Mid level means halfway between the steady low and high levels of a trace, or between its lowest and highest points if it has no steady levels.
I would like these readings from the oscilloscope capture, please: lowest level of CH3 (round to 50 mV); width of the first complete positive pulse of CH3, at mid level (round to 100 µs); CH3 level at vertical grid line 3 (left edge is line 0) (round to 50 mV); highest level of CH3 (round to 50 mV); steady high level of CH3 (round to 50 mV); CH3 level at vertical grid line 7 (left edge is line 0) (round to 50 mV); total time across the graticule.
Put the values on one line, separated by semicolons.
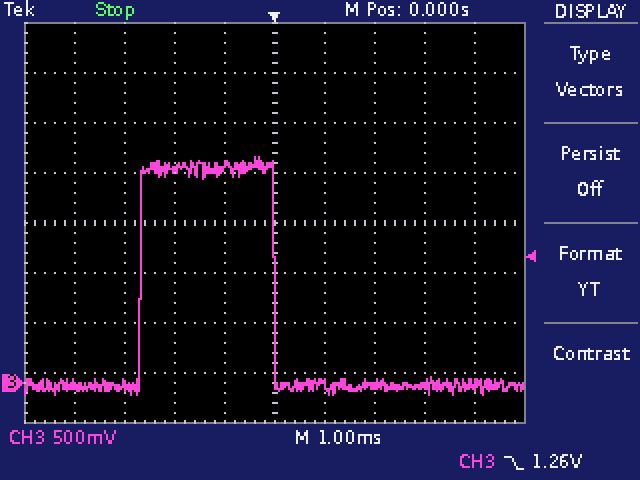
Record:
-100 mV; 2.7 ms; 2.15 V; 2.25 V; 2.15 V; 0 mV; 10 ms
